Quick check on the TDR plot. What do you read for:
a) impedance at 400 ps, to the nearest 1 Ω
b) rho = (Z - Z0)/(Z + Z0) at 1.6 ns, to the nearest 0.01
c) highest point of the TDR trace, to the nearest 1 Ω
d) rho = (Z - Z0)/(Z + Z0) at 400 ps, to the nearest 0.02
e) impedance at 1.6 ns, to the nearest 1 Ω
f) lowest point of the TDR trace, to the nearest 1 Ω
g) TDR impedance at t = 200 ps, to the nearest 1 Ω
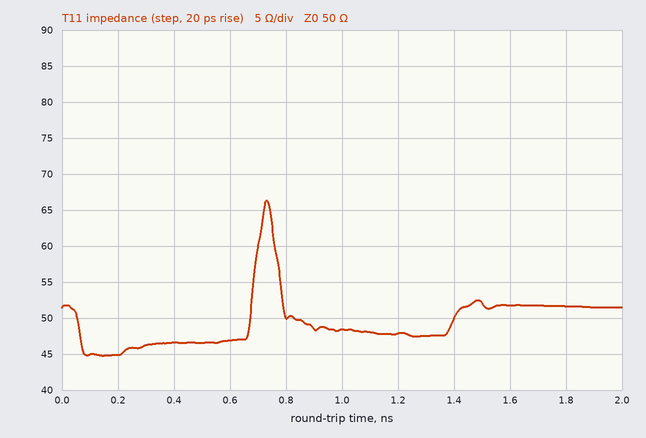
47 Ω
+0.02
66 Ω
-0.04
52 Ω
45 Ω
45 Ω
